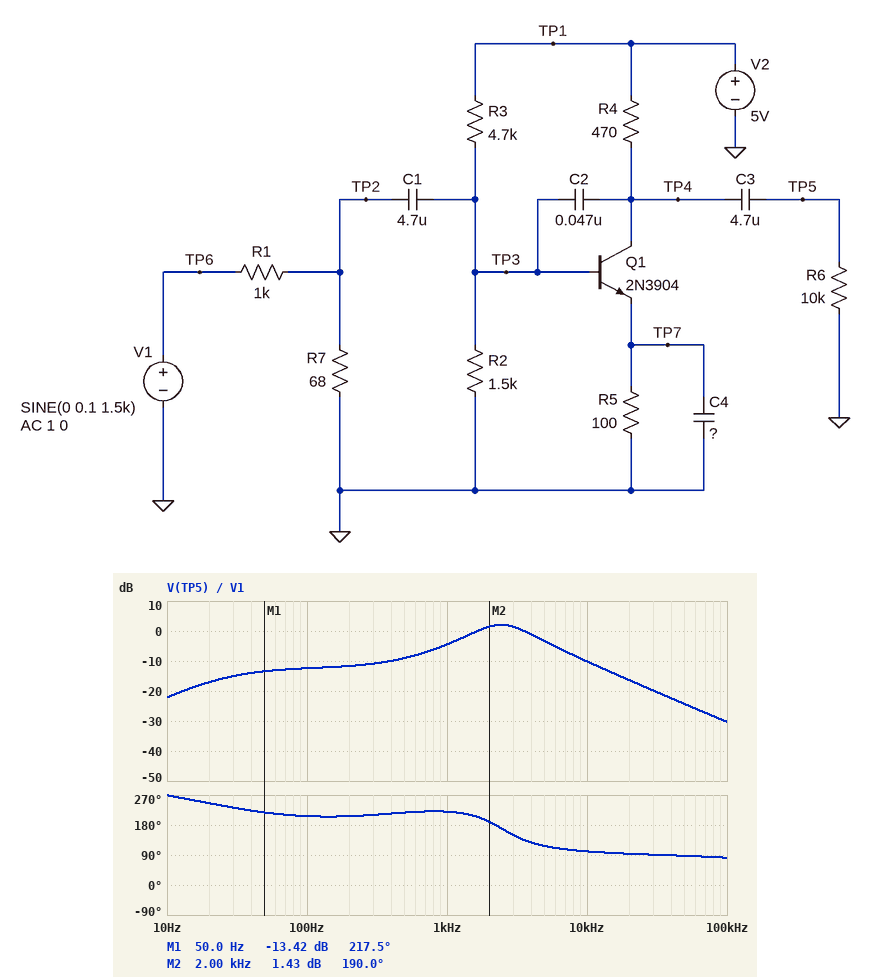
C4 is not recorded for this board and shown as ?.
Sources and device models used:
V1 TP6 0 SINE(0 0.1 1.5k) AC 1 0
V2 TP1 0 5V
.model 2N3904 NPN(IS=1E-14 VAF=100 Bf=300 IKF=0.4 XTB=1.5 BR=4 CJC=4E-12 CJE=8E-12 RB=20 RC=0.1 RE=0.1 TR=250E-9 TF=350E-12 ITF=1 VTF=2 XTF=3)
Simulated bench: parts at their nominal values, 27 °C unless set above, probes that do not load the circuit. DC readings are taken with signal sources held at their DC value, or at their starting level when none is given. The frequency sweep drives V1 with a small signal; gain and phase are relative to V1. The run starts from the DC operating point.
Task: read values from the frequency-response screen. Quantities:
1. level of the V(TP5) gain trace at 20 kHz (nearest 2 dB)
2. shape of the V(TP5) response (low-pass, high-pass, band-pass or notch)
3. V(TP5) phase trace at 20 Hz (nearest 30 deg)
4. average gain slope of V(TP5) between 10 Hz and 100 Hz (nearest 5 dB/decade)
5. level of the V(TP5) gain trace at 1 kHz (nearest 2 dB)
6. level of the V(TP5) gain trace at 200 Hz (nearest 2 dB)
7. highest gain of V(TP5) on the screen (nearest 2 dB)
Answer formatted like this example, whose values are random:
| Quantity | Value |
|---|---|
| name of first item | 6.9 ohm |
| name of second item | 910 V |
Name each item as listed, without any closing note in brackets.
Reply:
| Quantity | Value |
|---|---|
| level of the V(TP5) gain trace at 20 kHz | -16 dB |
| shape of the V(TP5) response | band-pass |
| V(TP5) phase trace at 20 Hz | 240 deg |
| average gain slope of V(TP5) between 10 Hz and 100 Hz | 10 dB/decade |
| level of the V(TP5) gain trace at 1 kHz | -4 dB |
| level of the V(TP5) gain trace at 200 Hz | -12 dB |
| highest gain of V(TP5) on the screen | 2 dB |
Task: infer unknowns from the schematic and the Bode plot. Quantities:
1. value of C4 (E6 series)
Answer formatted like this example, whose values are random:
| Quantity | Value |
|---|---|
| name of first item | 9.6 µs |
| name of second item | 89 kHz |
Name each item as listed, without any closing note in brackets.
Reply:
| Quantity | Value |
|---|---|
| value of C4 | 3.3 µF |
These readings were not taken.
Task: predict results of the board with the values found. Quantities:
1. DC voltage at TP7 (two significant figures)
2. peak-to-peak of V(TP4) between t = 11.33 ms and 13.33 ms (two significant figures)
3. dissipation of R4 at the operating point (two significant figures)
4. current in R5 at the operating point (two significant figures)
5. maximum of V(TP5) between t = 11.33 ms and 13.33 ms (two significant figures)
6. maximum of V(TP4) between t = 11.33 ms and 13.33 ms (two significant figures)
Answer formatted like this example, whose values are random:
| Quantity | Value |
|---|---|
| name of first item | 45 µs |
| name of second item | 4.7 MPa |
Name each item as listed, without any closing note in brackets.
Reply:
| Quantity | Value |
|---|---|
| DC voltage at TP7 | 490 mV |
| peak-to-peak of V(TP4) between t = 11.33 ms and 13.33 ms | 180 mV |
| dissipation of R4 at the operating point | 11 mW |
| current in R5 at the operating point | 4.9 mA |
| maximum of V(TP5) between t = 11.33 ms and 13.33 ms | 90 mV |
| maximum of V(TP4) between t = 11.33 ms and 13.33 ms | 2.8 V |
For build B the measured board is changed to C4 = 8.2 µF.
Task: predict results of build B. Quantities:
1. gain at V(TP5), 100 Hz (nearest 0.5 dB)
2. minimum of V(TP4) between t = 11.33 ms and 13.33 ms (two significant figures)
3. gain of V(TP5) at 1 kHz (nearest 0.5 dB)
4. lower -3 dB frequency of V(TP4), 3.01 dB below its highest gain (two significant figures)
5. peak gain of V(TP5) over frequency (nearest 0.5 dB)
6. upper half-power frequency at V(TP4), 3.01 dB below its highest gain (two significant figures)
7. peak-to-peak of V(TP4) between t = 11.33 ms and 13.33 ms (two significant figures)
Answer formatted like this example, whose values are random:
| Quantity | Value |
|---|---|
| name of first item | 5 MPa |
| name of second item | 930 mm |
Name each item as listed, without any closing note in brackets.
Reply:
| Quantity | Value |
|---|---|
| gain at V(TP5), 100 Hz | -11.5 dB |
| minimum of V(TP4) between t = 11.33 ms and 13.33 ms | 2.5 V |
| gain of V(TP5) at 1 kHz | 3.0 dB |
| lower -3 dB frequency of V(TP4), 3.01 dB below its highest gain | 930 Hz |
| peak gain of V(TP5) over frequency | 5.5 dB |
| upper half-power frequency at V(TP4), 3.01 dB below its highest gain | 2.6 kHz |
| peak-to-peak of V(TP4) between t = 11.33 ms and 13.33 ms | 370 mV |
